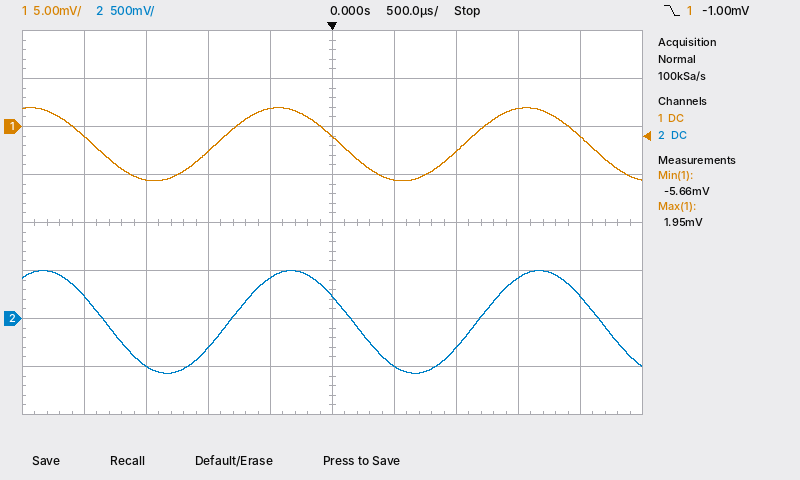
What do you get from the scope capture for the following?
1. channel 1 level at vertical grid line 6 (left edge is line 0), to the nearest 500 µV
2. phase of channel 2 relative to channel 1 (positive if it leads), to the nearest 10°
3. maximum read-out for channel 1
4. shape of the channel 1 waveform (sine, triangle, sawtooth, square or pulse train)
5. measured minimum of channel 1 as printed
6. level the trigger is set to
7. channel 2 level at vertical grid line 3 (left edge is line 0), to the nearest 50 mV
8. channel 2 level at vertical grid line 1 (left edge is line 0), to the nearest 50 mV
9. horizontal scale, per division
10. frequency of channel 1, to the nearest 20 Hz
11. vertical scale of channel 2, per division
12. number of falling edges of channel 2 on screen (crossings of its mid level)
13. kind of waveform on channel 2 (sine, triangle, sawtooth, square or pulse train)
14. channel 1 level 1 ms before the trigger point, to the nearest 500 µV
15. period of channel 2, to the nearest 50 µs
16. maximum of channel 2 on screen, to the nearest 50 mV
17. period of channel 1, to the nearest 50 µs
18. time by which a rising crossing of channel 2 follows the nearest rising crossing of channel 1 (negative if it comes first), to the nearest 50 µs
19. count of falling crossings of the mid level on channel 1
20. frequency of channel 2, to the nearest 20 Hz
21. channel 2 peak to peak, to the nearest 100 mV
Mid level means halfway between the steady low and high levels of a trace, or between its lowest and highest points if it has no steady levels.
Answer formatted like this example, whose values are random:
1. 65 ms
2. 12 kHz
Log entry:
1. -5.5 mV
2. -20°
3. 1.95 mV
4. sine
5. -5.66 mV
6. -1.00 mV
7. -300 mV
8. 250 mV
9. 500 µs
10. 500 Hz
11. 500 mV
12. 3
13. sine
14. -2.5 mV
15. 2.00 ms
16. 500 mV
17. 2.00 ms
18. +100 µs
19. 3
20. 500 Hz
21. 1.10 V
